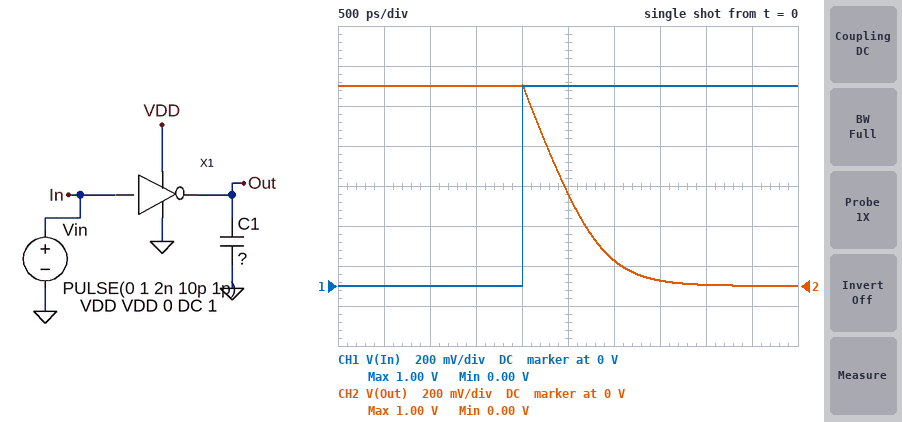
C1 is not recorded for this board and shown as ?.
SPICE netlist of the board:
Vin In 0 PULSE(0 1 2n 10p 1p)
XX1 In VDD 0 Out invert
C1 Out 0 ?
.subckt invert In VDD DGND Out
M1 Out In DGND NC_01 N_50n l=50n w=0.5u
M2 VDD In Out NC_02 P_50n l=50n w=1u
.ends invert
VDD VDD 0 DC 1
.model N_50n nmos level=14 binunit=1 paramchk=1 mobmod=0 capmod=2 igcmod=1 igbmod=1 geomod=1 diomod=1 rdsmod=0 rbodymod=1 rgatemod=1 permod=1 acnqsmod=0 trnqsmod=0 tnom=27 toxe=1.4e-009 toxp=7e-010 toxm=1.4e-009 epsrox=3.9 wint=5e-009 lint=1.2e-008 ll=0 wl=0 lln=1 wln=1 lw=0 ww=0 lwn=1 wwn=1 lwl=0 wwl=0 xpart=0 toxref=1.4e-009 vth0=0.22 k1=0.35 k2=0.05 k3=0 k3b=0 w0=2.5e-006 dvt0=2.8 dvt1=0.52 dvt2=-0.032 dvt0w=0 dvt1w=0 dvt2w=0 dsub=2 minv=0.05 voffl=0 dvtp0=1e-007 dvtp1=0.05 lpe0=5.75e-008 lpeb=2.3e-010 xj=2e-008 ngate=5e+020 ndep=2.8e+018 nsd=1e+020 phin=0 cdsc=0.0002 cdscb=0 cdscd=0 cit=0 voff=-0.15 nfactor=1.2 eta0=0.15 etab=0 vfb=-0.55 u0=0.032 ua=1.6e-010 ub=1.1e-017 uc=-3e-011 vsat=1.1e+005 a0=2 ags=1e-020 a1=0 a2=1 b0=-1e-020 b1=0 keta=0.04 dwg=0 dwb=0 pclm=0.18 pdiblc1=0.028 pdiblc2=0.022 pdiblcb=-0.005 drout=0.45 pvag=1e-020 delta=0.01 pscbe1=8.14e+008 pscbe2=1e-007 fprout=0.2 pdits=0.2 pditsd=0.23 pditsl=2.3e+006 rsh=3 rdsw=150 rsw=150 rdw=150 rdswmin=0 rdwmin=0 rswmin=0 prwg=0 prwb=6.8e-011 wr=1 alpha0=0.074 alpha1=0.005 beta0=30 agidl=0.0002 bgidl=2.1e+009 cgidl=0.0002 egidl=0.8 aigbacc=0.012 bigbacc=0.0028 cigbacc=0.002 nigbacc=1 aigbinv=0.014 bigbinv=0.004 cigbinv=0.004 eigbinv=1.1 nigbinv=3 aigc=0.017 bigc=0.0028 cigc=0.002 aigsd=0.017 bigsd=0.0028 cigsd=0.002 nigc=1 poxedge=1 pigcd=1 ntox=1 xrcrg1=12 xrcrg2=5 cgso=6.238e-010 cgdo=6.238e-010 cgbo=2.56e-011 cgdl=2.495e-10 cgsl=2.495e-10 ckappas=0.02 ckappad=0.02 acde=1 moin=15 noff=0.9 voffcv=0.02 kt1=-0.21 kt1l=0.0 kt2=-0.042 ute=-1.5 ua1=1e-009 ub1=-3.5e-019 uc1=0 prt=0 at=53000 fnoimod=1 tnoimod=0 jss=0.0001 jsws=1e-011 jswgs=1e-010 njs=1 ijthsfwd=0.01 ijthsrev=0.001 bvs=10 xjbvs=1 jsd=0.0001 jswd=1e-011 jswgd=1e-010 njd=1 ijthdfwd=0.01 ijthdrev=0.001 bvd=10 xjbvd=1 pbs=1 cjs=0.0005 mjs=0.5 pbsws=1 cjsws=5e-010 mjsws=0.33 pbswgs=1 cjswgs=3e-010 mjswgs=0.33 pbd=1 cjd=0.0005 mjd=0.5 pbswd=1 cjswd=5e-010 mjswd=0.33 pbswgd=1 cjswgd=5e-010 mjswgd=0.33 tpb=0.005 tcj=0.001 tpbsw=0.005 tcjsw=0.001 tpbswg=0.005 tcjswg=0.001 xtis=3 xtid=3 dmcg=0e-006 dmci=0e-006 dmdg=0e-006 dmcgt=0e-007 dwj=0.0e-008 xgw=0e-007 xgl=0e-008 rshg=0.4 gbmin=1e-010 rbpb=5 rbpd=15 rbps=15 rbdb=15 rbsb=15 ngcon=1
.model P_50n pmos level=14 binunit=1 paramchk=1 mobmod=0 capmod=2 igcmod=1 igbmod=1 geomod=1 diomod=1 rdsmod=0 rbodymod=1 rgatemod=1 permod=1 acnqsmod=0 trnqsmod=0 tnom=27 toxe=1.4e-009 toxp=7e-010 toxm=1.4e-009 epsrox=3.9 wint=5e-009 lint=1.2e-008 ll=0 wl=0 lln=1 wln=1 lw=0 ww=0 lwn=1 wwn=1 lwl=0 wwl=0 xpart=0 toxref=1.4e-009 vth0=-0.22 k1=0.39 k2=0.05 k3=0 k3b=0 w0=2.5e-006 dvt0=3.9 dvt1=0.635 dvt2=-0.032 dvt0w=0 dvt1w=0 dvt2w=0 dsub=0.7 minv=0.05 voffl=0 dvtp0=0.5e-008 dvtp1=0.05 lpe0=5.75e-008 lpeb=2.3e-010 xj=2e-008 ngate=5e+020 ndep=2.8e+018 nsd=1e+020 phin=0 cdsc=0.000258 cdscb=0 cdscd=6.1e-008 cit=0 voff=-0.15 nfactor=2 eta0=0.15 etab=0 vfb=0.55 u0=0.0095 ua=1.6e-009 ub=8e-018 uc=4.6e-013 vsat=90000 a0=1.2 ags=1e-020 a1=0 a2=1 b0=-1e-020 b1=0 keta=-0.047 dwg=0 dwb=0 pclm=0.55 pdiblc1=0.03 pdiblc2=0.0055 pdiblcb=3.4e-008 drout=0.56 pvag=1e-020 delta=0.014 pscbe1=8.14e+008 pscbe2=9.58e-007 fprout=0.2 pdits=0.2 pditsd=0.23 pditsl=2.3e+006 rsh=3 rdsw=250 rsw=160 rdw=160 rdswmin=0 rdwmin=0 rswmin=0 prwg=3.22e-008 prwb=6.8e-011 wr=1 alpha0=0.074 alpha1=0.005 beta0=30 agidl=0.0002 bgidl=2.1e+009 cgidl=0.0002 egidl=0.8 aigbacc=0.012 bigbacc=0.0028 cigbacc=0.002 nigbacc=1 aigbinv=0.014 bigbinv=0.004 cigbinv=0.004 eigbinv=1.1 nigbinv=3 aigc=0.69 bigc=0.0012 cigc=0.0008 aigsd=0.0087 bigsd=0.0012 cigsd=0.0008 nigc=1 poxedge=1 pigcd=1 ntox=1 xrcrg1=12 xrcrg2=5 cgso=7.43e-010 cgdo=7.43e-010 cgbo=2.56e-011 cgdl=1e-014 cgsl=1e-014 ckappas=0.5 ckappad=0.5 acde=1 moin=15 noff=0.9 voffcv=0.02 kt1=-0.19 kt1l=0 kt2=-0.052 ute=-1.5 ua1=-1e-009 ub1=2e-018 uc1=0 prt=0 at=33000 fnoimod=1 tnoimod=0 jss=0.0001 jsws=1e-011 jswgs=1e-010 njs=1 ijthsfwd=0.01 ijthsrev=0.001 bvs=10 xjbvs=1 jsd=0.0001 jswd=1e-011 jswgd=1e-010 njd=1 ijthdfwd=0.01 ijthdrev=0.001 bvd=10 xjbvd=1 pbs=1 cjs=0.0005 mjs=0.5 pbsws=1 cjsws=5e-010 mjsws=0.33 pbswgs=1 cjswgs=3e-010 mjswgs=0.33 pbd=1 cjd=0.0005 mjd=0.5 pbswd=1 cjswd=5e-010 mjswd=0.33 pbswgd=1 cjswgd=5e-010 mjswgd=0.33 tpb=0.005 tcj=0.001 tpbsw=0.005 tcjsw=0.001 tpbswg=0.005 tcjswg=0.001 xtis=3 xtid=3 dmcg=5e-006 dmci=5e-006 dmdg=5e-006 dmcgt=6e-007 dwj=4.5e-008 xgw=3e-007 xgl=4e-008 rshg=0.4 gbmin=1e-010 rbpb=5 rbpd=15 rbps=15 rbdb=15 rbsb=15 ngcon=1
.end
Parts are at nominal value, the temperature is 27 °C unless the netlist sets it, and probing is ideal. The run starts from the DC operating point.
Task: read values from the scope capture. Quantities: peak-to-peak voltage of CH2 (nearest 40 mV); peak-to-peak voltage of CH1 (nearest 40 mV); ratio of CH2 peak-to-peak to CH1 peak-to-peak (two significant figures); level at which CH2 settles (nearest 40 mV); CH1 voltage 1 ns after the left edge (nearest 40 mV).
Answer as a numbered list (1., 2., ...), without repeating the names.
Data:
1. 1.00 V
2. 1.00 V
3. 1.0
4. 0 V
5. 0 V
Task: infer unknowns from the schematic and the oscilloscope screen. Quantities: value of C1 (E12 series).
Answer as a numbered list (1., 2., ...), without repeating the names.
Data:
1. 270 fF
